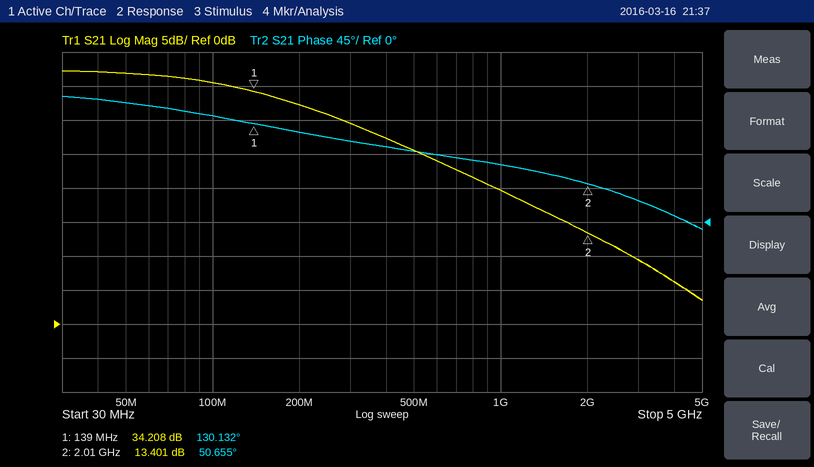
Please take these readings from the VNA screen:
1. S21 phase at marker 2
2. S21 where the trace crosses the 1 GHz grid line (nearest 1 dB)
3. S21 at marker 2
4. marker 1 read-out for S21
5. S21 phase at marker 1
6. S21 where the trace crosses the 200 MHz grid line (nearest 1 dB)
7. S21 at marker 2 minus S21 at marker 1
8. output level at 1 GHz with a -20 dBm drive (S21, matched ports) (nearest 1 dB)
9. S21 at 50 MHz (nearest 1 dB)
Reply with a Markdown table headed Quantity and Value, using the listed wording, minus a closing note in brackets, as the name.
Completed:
| Quantity | Value |
|---|---|
| S21 phase at marker 2 | 50.655° |
| S21 where the trace crosses the 1 GHz grid line | 20 dB |
| S21 at marker 2 | 13.401 dB |
| marker 1 read-out for S21 | 34.208 dB |
| S21 phase at marker 1 | 130.132° |
| S21 where the trace crosses the 200 MHz grid line | 32 dB |
| S21 at marker 2 minus S21 at marker 1 | -20.807 dB |
| output level at 1 GHz with a -20 dBm drive (S21, matched ports) | 0 dBm |
| S21 at 50 MHz | 37 dB |
